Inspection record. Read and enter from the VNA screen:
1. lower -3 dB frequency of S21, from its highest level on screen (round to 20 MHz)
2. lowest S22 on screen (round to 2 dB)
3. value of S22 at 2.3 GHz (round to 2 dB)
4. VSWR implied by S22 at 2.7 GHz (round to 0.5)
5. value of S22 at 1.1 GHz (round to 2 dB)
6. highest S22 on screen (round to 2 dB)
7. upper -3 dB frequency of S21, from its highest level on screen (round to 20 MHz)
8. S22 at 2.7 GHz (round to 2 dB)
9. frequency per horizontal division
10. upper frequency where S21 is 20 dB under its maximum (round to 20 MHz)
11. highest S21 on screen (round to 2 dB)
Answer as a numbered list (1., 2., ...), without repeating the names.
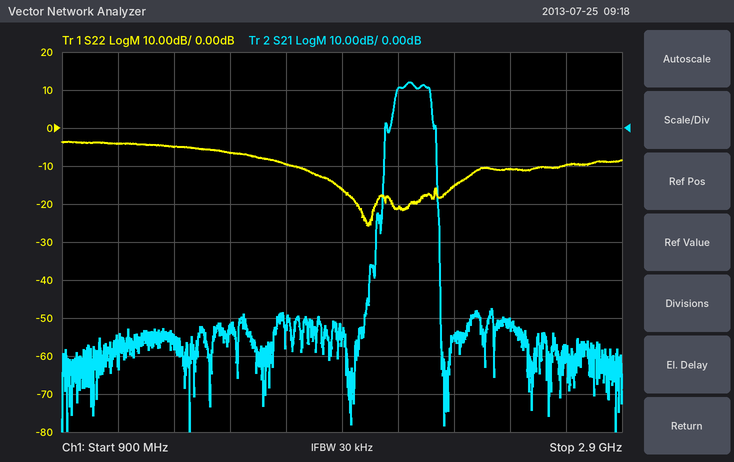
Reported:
1. 2.10 GHz
2. -26 dB
3. -16 dB
4. 2.0
5. -4 dB
6. -4 dB
7. 2.22 GHz
8. -10 dB
9. 200 MHz
10. 2.24 GHz
11. 12 dB
